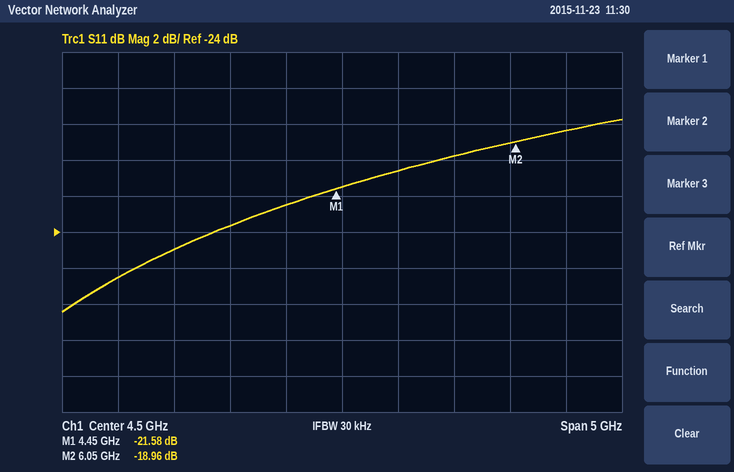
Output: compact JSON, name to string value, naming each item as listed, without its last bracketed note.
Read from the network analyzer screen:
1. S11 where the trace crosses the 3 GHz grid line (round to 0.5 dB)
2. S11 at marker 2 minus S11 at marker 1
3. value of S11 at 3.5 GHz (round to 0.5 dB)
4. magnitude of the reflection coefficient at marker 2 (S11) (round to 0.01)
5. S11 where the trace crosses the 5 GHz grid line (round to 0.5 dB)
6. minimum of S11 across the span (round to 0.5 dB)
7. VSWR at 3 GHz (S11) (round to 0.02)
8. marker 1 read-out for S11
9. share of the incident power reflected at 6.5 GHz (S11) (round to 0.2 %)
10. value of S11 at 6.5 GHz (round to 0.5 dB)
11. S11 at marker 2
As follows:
{"S11 where the trace crosses the 3 GHz grid line": "-25.0 dB", "S11 at marker 2 minus S11 at marker 1": "2.62 dB", "value of S11 at 3.5 GHz": "-23.5 dB", "magnitude of the reflection coefficient at marker 2 (S11)": "0.11", "S11 where the trace crosses the 5 GHz grid line": "-20.5 dB", "minimum of S11 across the span": "-28.5 dB", "VSWR at 3 GHz (S11)": "1.12", "marker 1 read-out for S11": "-21.58 dB", "share of the incident power reflected at 6.5 GHz (S11)": "1.4 %", "value of S11 at 6.5 GHz": "-18.5 dB", "S11 at marker 2": "-18.96 dB"}
